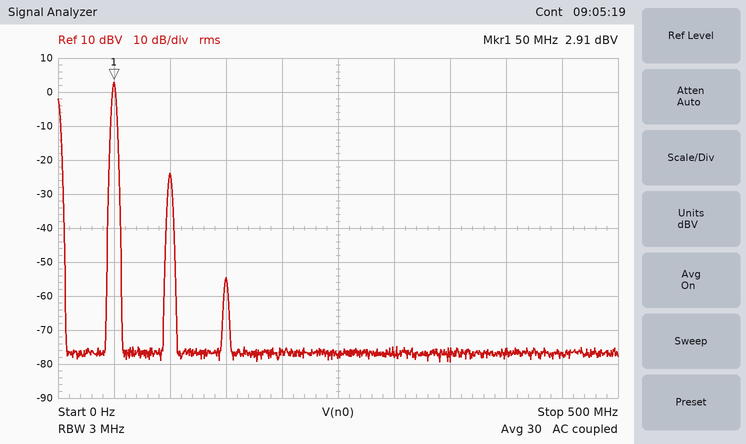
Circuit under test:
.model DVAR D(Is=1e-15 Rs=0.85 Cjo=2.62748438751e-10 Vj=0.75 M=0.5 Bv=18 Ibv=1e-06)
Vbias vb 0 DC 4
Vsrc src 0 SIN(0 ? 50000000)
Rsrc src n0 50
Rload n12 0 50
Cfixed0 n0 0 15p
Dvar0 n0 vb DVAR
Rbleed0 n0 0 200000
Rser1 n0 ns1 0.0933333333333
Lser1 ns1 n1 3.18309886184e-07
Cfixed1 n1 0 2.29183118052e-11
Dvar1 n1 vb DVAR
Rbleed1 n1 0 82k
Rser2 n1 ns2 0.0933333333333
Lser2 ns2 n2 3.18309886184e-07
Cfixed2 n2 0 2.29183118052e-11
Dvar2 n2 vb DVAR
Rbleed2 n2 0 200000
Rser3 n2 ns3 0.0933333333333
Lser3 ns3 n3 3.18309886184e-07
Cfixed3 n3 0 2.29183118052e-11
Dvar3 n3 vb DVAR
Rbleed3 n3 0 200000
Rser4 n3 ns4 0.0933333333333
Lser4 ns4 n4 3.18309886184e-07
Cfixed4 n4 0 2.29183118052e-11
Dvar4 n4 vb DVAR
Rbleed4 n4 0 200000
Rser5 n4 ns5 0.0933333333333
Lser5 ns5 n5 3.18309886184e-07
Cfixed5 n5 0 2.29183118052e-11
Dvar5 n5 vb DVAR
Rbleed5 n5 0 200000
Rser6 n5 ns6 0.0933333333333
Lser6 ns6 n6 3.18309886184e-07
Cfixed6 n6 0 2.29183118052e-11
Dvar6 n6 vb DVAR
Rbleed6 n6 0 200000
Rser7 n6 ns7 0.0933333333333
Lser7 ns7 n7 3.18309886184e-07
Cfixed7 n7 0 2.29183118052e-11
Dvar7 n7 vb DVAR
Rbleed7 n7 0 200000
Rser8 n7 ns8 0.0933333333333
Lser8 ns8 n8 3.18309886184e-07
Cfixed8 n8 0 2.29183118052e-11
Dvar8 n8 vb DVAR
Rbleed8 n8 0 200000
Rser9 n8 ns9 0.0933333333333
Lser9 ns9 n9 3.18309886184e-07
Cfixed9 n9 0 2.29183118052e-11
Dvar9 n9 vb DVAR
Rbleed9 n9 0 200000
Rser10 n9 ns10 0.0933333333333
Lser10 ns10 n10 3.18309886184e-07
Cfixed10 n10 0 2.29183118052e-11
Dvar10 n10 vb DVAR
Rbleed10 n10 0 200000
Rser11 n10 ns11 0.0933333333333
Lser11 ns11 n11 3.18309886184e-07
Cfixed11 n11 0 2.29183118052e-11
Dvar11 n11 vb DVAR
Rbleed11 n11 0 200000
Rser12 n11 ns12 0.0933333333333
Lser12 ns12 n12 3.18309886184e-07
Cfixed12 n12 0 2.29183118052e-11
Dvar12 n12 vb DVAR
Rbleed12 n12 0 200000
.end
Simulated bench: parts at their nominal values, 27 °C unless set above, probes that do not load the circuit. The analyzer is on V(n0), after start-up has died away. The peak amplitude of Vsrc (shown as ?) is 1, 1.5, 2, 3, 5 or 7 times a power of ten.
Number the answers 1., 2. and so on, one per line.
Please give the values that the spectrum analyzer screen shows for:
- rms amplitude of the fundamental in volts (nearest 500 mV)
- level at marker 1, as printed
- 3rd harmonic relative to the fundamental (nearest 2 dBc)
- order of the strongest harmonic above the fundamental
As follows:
1. 1.5 V
2. 2.91 dBV
3. -58 dBc
4. 2
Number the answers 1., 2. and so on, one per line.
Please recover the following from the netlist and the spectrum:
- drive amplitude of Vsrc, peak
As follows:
1. 3 V
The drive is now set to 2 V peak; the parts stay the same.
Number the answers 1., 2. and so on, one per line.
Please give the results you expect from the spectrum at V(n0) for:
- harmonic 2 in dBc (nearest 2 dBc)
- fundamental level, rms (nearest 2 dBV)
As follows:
1. -30 dBc
2. 0 dBV
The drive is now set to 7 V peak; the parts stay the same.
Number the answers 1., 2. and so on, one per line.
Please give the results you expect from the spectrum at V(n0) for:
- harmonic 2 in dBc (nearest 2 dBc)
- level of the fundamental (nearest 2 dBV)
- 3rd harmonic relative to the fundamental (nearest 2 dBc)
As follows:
1. -18 dBc
2. 10 dBV
3. -42 dBc
